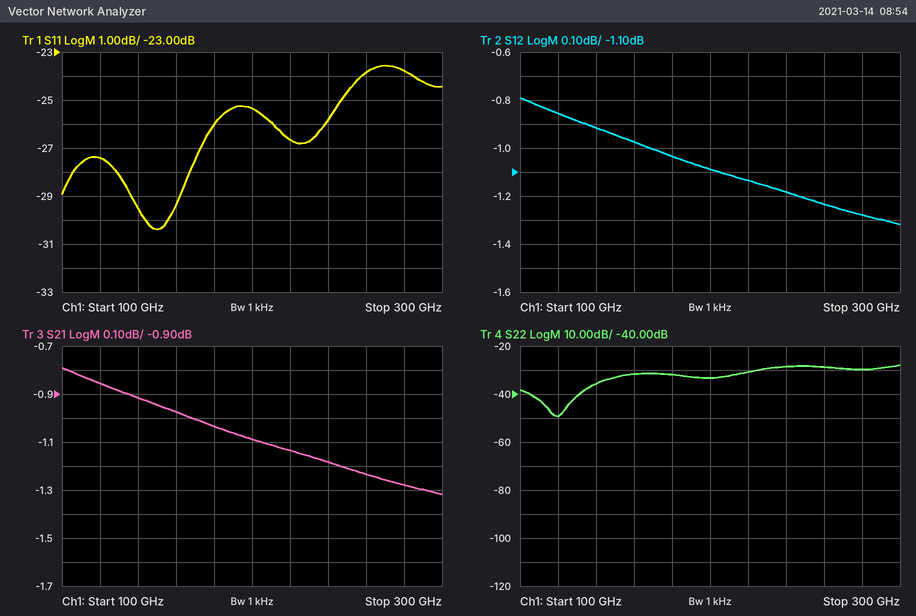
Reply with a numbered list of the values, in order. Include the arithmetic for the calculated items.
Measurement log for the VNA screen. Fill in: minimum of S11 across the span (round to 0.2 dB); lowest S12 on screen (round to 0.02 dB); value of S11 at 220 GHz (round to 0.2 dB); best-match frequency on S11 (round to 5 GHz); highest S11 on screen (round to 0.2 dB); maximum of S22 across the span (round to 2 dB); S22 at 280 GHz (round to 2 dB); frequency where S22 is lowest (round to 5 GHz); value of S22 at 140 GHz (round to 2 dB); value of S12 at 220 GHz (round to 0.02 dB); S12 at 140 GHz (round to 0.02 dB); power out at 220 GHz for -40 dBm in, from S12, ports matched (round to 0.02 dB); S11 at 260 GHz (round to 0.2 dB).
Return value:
1. -30.4 dB
2. -1.32 dB
3. -26.6 dB
4. 150 GHz
5. -23.6 dB
6. -28 dB
7. -30 dB
8. 120 GHz
9. -36 dB
10. -1.14 dB
11. -0.92 dB
12. -40 dBm + (-1.14 dB) = -41.14 dBm
13. -23.8 dB
